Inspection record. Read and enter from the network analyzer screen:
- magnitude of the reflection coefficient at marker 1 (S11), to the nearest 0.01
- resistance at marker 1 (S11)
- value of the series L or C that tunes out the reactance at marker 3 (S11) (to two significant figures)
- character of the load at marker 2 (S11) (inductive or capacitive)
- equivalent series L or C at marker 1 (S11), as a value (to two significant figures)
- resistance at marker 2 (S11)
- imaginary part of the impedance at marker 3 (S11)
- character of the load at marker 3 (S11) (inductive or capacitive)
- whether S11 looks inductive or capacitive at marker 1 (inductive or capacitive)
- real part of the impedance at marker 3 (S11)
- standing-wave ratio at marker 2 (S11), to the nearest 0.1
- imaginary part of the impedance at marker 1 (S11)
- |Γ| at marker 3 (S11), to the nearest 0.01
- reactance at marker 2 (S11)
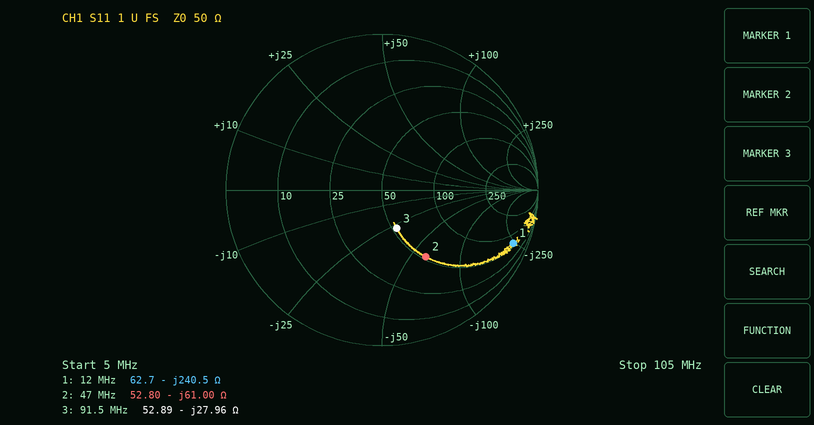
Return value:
0.91
62.7 Ω
49 nH
capacitive
55 pF
52.80 Ω
-27.96 Ω
capacitive
capacitive
52.89 Ω
3.1
-240.5 Ω
0.26
-61.00 Ω
